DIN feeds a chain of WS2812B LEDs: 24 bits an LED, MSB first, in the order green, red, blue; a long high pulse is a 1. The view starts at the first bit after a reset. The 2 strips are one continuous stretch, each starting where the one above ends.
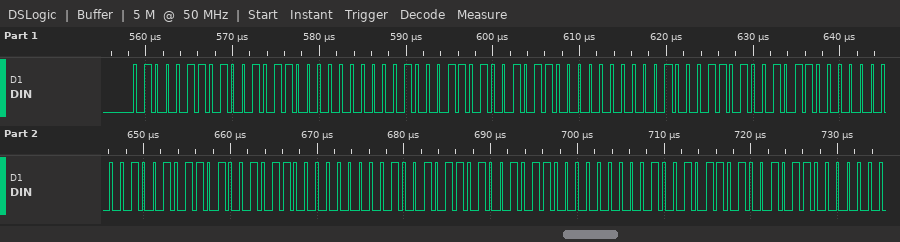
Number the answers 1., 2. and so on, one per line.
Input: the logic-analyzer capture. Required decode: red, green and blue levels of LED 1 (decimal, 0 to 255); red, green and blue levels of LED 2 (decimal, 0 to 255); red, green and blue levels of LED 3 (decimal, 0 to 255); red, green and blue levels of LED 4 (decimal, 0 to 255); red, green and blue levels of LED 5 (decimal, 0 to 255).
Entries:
1. 150, 70, 0
2. 150, 70, 0
3. 150, 70, 0
4. 150, 150, 0
5. 150, 150, 0
